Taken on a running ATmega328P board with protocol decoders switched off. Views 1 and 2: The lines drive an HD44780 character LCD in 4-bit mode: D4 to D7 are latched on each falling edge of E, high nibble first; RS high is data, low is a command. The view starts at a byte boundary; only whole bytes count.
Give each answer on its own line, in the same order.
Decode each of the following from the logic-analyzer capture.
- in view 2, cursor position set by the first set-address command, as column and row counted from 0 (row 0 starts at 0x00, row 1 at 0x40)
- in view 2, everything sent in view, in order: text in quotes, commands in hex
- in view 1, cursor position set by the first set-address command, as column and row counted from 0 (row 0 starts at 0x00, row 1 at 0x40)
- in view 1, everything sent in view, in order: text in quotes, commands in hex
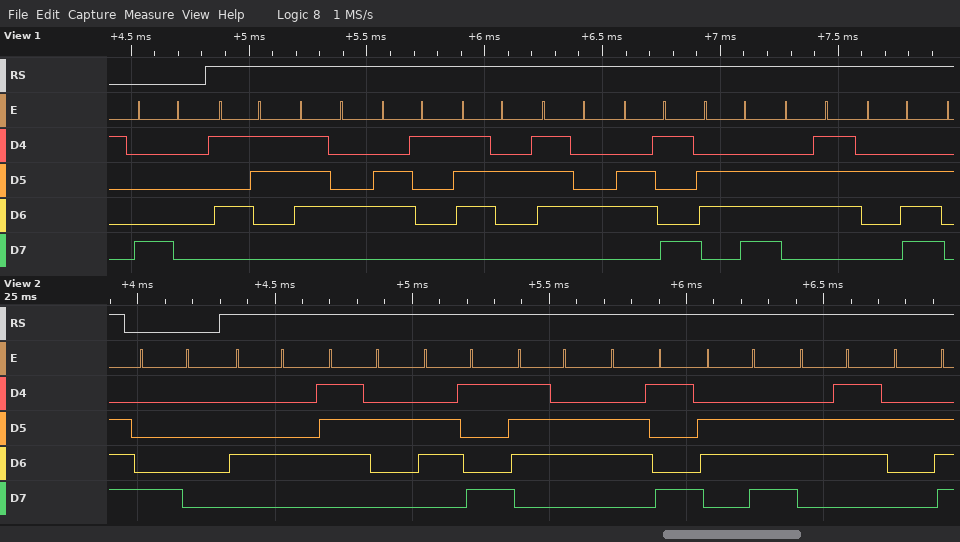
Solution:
column 0, row 0
0x80 "Driving."
column 0, row 0
0x80 "Starting."
